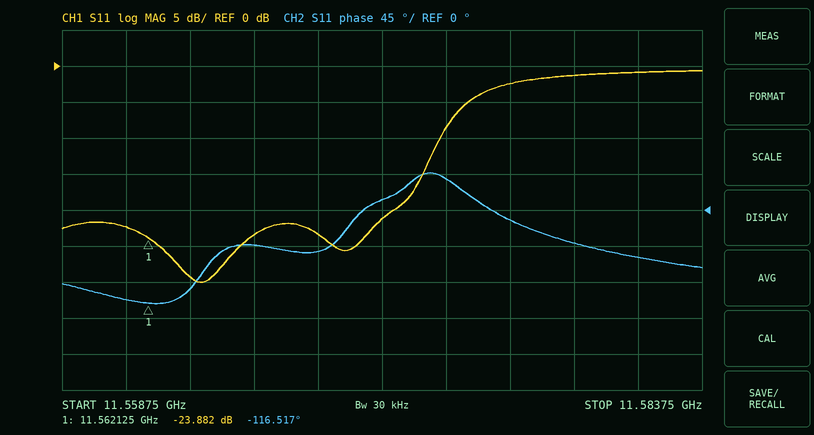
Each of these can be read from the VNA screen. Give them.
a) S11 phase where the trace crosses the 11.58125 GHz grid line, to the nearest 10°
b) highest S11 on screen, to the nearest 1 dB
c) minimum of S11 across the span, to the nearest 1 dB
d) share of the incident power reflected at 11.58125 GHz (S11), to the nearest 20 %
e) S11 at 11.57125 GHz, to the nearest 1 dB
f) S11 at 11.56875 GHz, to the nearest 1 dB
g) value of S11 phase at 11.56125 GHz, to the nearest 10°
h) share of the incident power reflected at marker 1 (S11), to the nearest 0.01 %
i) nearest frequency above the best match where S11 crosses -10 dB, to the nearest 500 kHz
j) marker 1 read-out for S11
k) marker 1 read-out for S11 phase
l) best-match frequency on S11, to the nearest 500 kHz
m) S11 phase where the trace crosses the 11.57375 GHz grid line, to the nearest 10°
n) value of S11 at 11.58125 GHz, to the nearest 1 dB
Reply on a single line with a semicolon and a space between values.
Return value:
-60°; -1 dB; -30 dB; 80 %; -21 dB; -23 dB; -110°; 0.41 %; 11.5735 GHz; -23.882 dB; -116.517°; 11.5640 GHz; 40°; -1 dB
